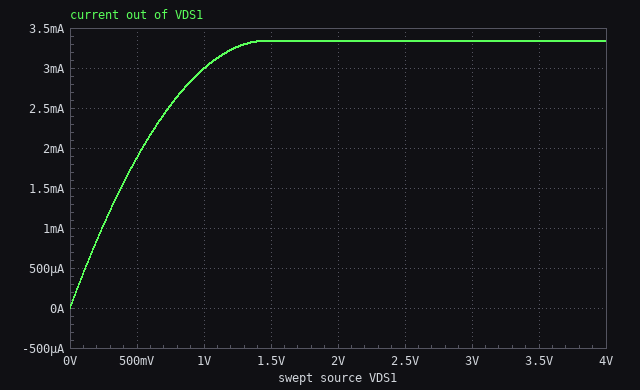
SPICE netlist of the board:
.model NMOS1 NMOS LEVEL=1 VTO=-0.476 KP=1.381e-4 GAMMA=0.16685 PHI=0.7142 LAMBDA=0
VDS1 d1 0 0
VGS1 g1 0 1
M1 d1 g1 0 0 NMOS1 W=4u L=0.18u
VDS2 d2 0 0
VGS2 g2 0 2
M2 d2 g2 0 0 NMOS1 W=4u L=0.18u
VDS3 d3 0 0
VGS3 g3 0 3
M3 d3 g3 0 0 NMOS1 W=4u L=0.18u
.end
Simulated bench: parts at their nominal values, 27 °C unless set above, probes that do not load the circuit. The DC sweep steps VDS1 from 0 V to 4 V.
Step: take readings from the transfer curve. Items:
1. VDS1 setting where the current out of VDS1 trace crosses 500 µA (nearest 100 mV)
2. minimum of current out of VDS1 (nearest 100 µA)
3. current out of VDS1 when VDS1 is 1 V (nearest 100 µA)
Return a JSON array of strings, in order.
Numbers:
["100 mV", "0 A", "3.0 mA"]
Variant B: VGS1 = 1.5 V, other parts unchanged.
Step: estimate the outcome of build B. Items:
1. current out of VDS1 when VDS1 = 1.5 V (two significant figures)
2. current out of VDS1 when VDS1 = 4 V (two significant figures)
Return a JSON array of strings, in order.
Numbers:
["5.6 mA", "6.0 mA"]
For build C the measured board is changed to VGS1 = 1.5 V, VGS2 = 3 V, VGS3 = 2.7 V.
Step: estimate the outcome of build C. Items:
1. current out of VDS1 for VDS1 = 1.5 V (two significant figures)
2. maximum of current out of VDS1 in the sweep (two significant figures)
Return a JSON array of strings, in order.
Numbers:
["5.6 mA", "6.0 mA"]
